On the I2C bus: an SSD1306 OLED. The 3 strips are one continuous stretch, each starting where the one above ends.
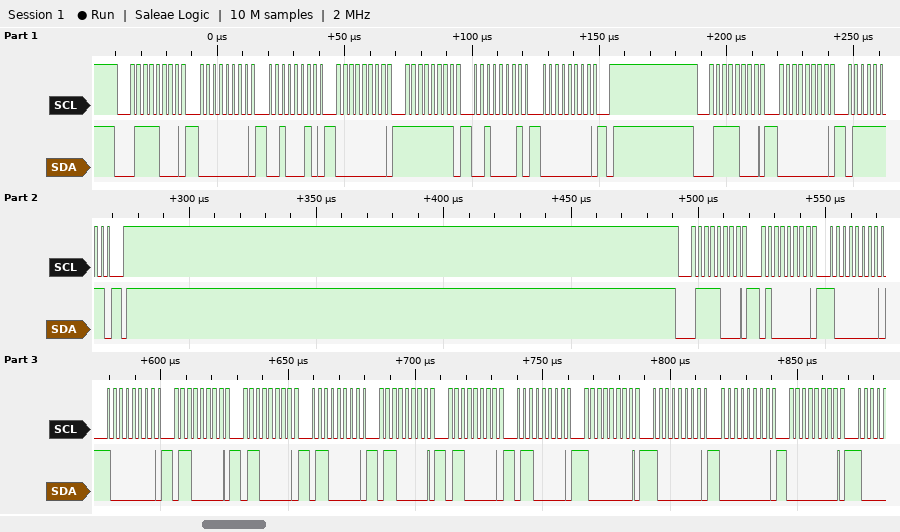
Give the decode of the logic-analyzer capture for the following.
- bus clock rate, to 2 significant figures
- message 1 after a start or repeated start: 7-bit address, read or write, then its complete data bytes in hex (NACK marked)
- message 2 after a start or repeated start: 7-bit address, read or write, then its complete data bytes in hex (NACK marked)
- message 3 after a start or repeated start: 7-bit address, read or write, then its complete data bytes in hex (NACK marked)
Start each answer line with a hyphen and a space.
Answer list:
- 400 kHz
- 0x3C write: 00 22 00 FF 21 00
- 0x3C write: 00 7F
- 0x3C write: 40 80 80 60 60 60 60 60 60 80 80 00 00
